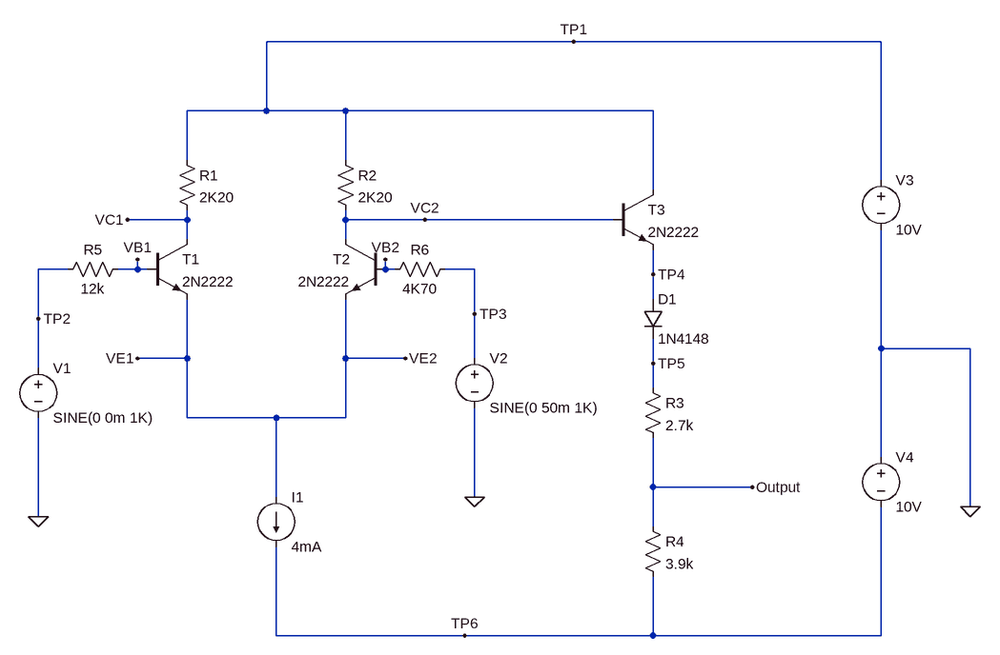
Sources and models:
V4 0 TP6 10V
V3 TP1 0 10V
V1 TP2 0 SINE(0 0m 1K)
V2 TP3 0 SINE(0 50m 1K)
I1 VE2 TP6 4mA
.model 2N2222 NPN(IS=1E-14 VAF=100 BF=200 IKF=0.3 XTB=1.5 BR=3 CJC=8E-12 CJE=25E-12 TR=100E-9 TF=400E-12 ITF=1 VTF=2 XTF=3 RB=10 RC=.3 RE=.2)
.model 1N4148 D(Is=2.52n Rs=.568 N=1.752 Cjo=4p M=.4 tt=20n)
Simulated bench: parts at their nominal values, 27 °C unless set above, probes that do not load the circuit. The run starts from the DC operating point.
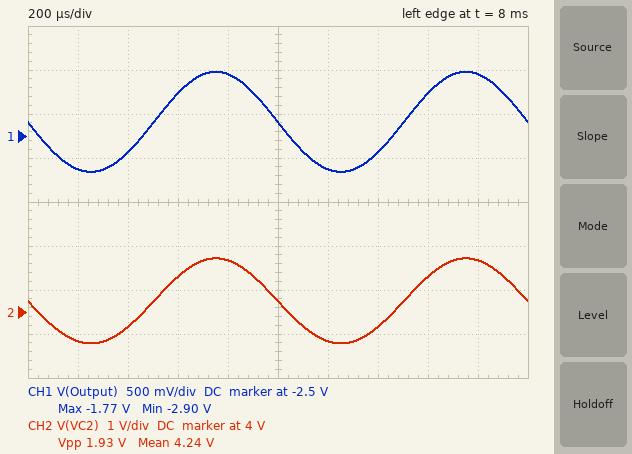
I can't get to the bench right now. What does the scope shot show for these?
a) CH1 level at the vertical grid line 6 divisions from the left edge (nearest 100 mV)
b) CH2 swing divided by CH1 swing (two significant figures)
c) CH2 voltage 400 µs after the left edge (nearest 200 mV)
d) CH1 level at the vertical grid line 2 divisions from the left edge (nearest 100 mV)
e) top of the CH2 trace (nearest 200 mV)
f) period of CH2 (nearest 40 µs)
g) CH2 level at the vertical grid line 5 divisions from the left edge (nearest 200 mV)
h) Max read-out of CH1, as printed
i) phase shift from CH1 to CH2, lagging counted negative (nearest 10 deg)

-2.9 V
1.7
3.6 V
-2.7 V
5.2 V
1.00 ms
4.2 V
-1.77 V
0 deg
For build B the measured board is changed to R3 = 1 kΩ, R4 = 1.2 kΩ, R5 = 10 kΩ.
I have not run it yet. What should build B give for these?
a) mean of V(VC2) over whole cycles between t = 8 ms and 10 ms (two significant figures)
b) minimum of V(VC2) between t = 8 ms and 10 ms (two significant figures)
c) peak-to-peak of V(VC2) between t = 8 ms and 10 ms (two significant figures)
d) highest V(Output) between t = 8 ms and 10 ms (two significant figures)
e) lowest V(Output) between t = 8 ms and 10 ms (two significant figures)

4.5 V
3.4 V
2.1 V
-2.3 V
-3.4 V
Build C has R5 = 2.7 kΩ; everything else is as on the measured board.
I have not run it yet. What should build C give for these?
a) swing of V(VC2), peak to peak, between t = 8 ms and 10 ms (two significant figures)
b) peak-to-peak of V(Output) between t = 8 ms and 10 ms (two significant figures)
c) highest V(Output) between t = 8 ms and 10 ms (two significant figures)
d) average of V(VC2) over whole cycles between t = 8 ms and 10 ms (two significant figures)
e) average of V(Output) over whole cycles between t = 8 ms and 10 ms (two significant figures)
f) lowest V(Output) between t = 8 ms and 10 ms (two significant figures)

3.3 V
1.9 V
-220 mV
6.2 V
-1.2 V
-2.2 V
